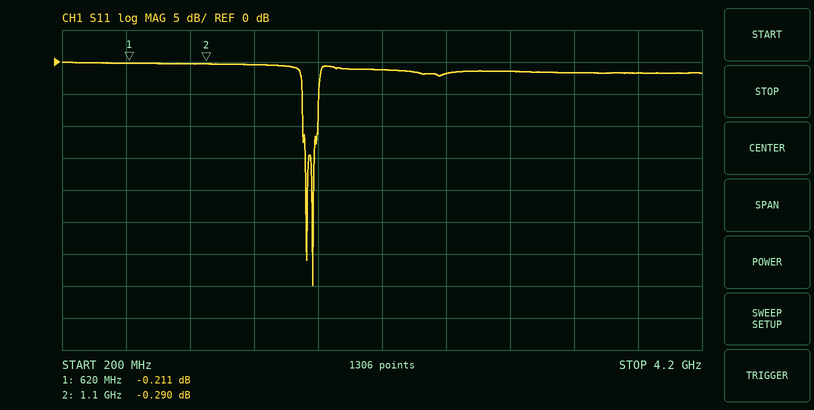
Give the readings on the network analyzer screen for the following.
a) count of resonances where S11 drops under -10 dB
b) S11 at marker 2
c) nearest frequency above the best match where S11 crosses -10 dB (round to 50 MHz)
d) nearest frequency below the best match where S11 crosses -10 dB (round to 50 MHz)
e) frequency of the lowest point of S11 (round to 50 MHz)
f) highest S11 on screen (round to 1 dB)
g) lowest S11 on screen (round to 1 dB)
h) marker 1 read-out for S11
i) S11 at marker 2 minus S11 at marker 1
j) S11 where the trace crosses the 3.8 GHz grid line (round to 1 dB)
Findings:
2
-0.290 dB
1.80 GHz
1.70 GHz
1.75 GHz
0 dB
-35 dB
-0.211 dB
-0.079 dB
-2 dB
